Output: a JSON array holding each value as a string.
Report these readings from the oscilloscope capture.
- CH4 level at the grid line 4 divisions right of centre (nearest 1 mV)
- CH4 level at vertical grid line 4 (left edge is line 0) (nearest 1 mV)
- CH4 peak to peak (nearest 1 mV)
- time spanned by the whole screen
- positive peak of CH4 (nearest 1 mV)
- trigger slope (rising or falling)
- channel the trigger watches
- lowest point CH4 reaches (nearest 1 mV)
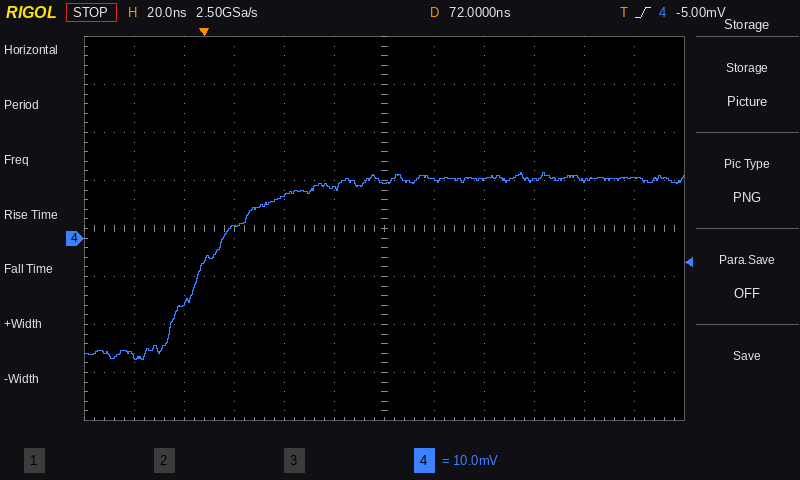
["12 mV", "9 mV", "39 mV", "240 ns", "14 mV", "rising", "CH4", "-25 mV"]
